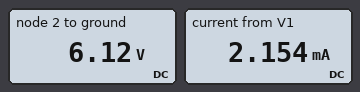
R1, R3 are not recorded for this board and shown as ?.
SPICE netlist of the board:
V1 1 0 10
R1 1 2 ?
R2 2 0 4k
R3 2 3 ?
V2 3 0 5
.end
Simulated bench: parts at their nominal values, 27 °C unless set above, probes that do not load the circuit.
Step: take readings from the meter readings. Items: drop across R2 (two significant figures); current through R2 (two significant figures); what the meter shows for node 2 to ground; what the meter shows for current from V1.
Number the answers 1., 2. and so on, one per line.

1. 6.1 V
2. 1.5 mA
3. 6.12 V
4. 2.154 mA
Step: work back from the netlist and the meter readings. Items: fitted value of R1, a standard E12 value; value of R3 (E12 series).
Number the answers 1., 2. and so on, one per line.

1. 1.8 kΩ
2. 1.8 kΩ
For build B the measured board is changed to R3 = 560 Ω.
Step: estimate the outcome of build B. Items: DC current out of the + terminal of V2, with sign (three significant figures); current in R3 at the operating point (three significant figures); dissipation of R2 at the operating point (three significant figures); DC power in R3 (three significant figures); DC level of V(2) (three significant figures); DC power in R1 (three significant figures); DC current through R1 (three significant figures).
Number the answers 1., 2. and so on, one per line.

1. -1.05 mA
2. 1.05 mA
3. 7.81 mW
4. 621 µW
5. 5.59 V
6. 10.8 mW
7. 2.45 mA
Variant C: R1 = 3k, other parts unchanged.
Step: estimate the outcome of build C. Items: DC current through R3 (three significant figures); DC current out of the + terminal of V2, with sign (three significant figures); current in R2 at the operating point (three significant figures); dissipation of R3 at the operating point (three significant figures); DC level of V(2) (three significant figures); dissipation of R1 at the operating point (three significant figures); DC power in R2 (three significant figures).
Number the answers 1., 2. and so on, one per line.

1. 203 µA
2. -203 µA
3. 1.34 mA
4. 74.4 µW
5. 5.37 V
6. 7.16 mW
7. 7.20 mW
